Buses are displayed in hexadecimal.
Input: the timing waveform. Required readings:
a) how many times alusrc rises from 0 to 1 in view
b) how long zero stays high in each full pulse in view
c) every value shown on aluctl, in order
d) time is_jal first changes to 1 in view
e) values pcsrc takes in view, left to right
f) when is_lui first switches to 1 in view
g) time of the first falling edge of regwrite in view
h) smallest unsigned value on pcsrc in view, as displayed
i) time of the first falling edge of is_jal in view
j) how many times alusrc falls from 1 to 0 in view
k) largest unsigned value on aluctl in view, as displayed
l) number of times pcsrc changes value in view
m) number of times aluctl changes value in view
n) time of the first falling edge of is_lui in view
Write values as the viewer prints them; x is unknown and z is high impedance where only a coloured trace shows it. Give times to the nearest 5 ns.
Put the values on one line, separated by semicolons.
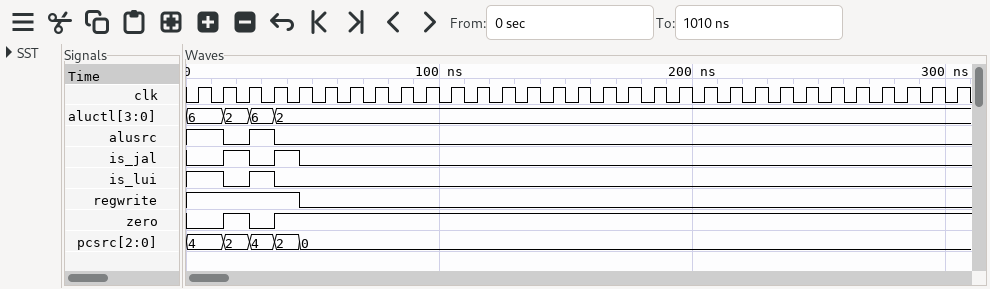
1; 10 ns; 6, 2, 6, 2; 15 ns; 4, 2, 4, 2, 0; 25 ns; 45 ns; 0; 25 ns; 2; 6; 4; 3; 15 ns
